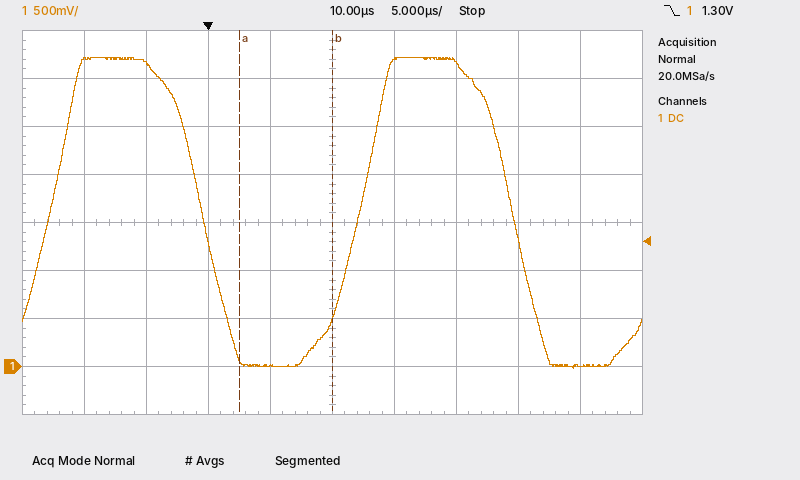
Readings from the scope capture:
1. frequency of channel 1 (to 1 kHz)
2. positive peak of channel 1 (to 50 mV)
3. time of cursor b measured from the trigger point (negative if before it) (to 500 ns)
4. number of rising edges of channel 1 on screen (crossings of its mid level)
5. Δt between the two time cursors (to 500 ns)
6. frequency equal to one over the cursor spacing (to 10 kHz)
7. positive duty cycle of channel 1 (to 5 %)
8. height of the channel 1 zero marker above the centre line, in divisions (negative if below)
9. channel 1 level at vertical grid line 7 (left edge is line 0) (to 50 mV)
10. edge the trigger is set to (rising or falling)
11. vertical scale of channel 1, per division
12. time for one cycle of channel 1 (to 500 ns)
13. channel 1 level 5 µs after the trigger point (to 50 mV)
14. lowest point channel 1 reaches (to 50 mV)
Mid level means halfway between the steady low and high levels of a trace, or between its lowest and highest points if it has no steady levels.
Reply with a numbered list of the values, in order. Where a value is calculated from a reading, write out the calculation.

1. 1 / 25.0 µs ≈ 40 kHz
2. 3.20 V
3. +10.0 µs
4. 2
5. 7.5 µs
6. 1 / 7.5 µs ≈ 130 kHz
7. 50 %
8. -3.0 div
9. 3.15 V
10. falling
11. 500 mV
12. 25.0 µs
13. 0 mV
14. 0 mV
